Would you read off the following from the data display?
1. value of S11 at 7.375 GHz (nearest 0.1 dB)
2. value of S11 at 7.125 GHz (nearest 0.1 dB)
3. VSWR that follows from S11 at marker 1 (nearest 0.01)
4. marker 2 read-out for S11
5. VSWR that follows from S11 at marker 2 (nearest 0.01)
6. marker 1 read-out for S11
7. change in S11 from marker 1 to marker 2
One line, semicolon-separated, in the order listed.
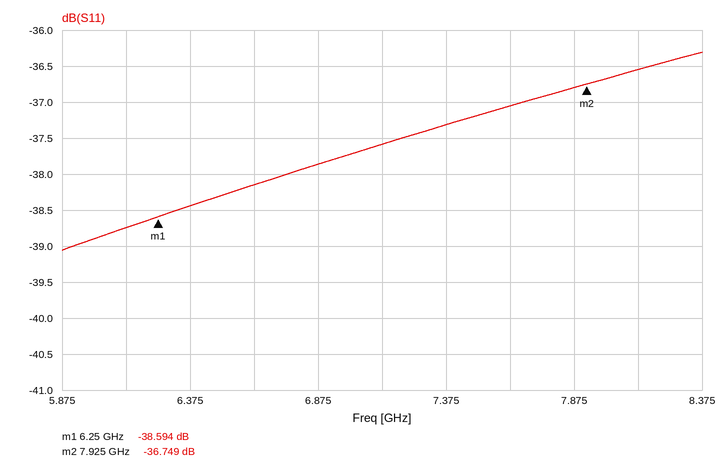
-37.3 dB; -37.6 dB; 1.02; -36.749 dB; 1.03; -38.594 dB; 1.845 dB
